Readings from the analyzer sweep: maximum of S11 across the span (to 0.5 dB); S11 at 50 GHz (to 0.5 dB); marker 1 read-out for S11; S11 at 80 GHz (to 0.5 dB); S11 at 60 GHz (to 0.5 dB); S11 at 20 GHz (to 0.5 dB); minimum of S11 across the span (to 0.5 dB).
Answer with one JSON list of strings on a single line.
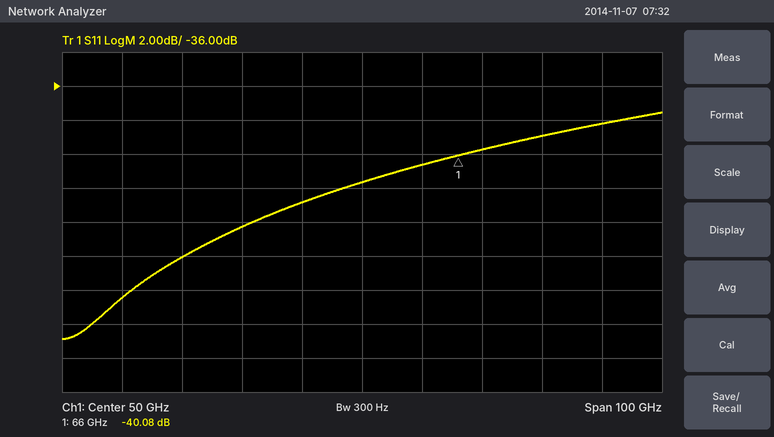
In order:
["-37.5 dB", "-41.5 dB", "-40.08 dB", "-39.0 dB", "-40.5 dB", "-46.0 dB", "-51.0 dB"]
